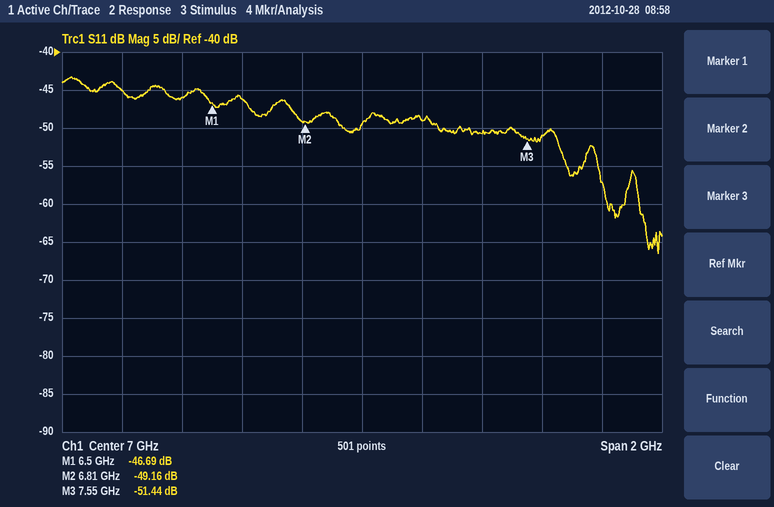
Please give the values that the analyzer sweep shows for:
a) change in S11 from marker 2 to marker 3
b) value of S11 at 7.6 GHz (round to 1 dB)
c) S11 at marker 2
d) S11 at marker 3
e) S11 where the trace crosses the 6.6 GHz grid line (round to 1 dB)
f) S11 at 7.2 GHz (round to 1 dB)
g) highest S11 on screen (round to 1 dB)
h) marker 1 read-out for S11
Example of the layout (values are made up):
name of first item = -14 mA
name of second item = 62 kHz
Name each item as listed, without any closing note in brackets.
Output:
change in S11 from marker 2 to marker 3 = -2.28 dB
value of S11 at 7.6 GHz = -51 dB
S11 at marker 2 = -49.16 dB
S11 at marker 3 = -51.44 dB
S11 where the trace crosses the 6.6 GHz grid line = -46 dB
S11 at 7.2 GHz = -49 dB
highest S11 on screen = -43 dB
marker 1 read-out for S11 = -46.69 dB
